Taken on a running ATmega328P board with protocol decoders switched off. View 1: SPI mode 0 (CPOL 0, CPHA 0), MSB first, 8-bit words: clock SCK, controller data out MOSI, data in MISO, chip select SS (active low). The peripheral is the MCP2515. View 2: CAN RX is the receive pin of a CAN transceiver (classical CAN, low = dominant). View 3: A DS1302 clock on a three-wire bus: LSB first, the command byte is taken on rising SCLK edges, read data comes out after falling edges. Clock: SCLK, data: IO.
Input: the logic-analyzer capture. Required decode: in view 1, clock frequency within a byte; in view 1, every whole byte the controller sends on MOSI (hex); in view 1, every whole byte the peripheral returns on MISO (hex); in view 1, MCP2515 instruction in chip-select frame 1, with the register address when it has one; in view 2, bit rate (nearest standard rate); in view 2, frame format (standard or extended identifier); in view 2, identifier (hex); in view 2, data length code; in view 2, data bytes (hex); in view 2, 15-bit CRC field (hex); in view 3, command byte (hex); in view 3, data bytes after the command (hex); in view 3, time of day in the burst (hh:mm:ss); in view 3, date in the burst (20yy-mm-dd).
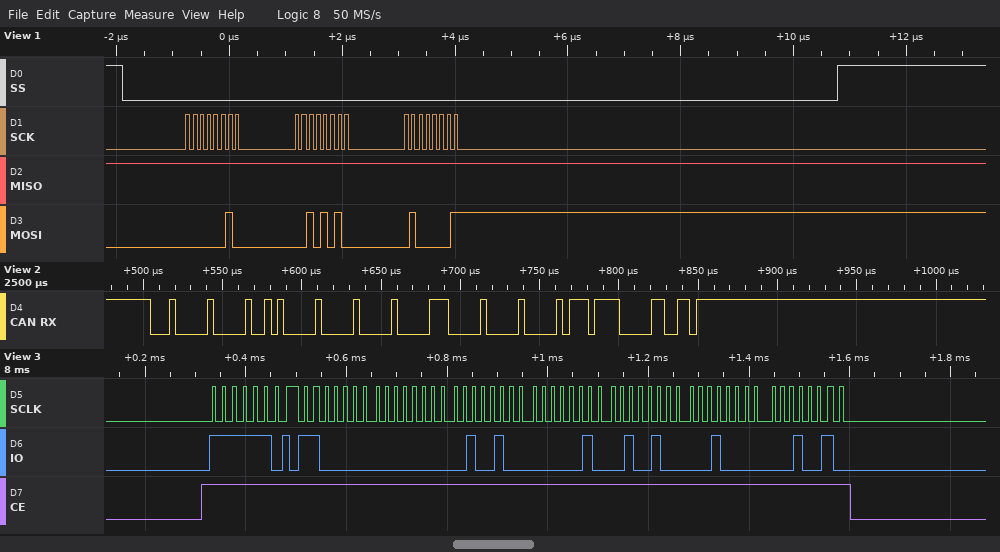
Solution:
8 MHz
0x02 0x2A 0x41
0xFF 0xFF 0xFF
WRITE 0x2A
250 kbit/s
standard
0x100
5
00 00 0C 00 03
0x5E09
0xBF
03 00 12 20 12 04 24
12:00:03
2024-12-20
